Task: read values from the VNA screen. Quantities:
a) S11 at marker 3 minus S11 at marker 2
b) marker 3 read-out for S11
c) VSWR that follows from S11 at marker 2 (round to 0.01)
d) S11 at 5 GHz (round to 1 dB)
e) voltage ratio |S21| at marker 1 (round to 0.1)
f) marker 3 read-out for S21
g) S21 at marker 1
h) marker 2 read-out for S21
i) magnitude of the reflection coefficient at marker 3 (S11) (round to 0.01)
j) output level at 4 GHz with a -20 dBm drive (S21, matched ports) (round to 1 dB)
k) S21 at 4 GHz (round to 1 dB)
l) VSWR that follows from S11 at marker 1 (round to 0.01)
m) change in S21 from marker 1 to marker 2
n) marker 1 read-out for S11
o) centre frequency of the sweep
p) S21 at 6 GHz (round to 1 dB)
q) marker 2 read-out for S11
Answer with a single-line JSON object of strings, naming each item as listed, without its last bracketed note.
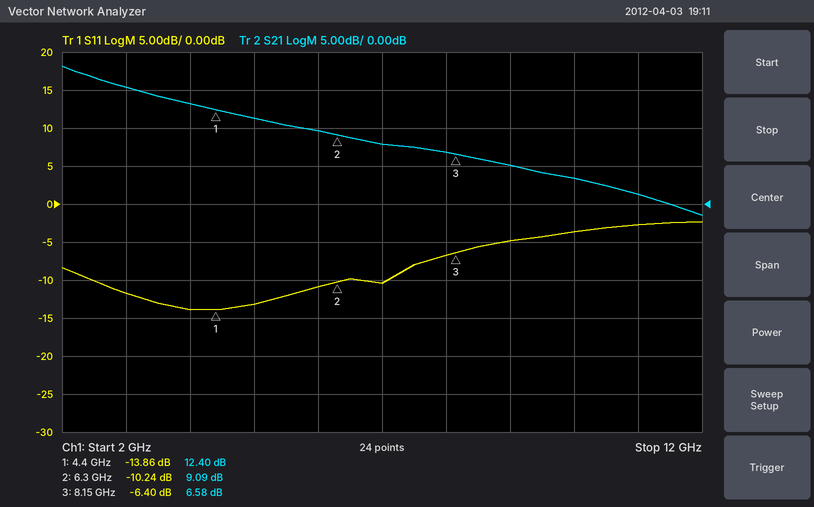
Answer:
{"S11 at marker 3 minus S11 at marker 2": "3.84 dB", "marker 3 read-out for S11": "-6.40 dB", "VSWR that follows from S11 at marker 2": "1.89", "S11 at 5 GHz": "-13 dB", "voltage ratio |S21| at marker 1": "4.2", "marker 3 read-out for S21": "6.58 dB", "S21 at marker 1": "12.40 dB", "marker 2 read-out for S21": "9.09 dB", "magnitude of the reflection coefficient at marker 3 (S11)": "0.48", "output level at 4 GHz with a -20 dBm drive (S21, matched ports)": "-7 dBm", "S21 at 4 GHz": "13 dB", "VSWR that follows from S11 at marker 1": "1.51", "change in S21 from marker 1 to marker 2": "-3.31 dB", "marker 1 read-out for S11": "-13.86 dB", "centre frequency of the sweep": "7 GHz", "S21 at 6 GHz": "10 dB", "marker 2 read-out for S11": "-10.24 dB"}
